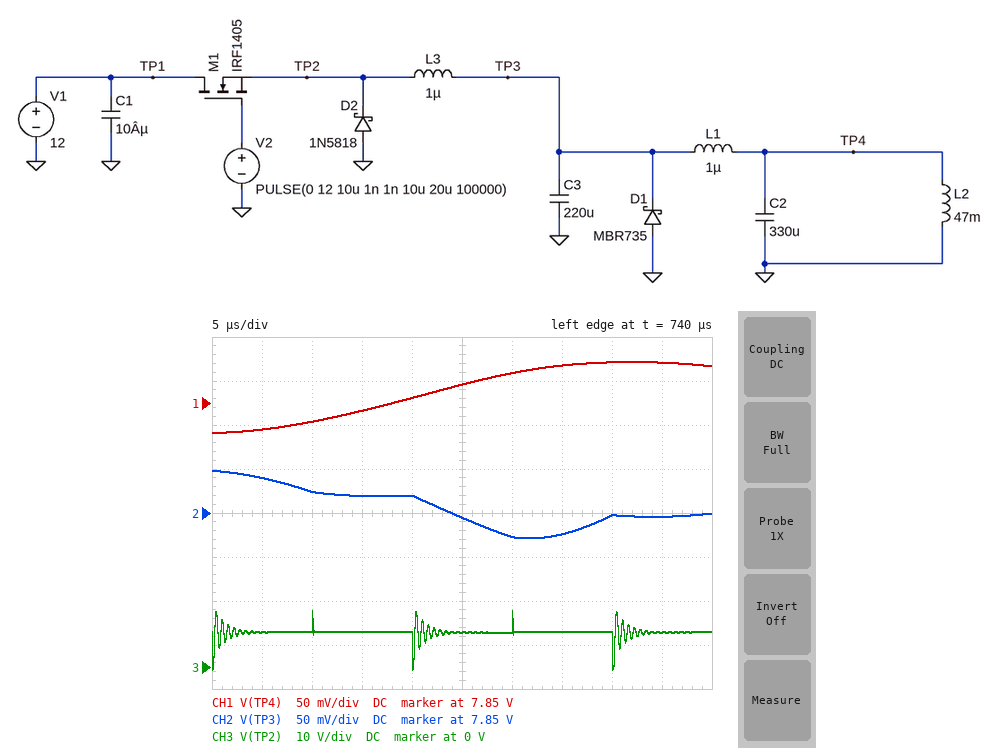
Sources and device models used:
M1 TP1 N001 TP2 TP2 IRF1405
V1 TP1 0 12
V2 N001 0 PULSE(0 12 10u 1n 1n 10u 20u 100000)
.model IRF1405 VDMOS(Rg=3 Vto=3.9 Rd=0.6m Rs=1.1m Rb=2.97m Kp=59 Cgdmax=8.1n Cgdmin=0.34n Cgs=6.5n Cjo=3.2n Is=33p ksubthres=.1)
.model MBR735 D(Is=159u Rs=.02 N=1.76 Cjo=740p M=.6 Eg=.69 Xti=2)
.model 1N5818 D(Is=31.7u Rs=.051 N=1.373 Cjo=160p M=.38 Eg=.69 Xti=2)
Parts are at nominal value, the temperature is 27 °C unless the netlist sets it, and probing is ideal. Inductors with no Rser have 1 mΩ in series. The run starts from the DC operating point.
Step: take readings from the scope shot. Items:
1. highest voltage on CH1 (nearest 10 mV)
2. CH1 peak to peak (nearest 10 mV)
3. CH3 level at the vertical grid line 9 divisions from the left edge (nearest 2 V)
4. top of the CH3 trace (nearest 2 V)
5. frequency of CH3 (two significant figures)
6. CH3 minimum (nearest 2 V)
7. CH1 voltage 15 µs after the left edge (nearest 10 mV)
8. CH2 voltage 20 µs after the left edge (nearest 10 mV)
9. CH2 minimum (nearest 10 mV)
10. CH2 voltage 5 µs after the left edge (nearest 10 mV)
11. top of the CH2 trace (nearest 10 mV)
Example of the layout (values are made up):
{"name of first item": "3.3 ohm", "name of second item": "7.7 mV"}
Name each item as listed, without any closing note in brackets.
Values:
{"highest voltage on CH1": "7.90 V", "CH1 peak to peak": "80 mV", "CH3 level at the vertical grid line 9 divisions from the left edge": "8 V", "top of the CH3 trace": "12 V", "frequency of CH3": "50 kHz", "CH3 minimum": "0 V", "CH1 voltage 15 µs after the left edge": "7.84 V", "CH2 voltage 20 µs after the left edge": "7.87 V", "CH2 minimum": "7.82 V", "CH2 voltage 5 µs after the left edge": "7.89 V", "top of the CH2 trace": "7.90 V"}
